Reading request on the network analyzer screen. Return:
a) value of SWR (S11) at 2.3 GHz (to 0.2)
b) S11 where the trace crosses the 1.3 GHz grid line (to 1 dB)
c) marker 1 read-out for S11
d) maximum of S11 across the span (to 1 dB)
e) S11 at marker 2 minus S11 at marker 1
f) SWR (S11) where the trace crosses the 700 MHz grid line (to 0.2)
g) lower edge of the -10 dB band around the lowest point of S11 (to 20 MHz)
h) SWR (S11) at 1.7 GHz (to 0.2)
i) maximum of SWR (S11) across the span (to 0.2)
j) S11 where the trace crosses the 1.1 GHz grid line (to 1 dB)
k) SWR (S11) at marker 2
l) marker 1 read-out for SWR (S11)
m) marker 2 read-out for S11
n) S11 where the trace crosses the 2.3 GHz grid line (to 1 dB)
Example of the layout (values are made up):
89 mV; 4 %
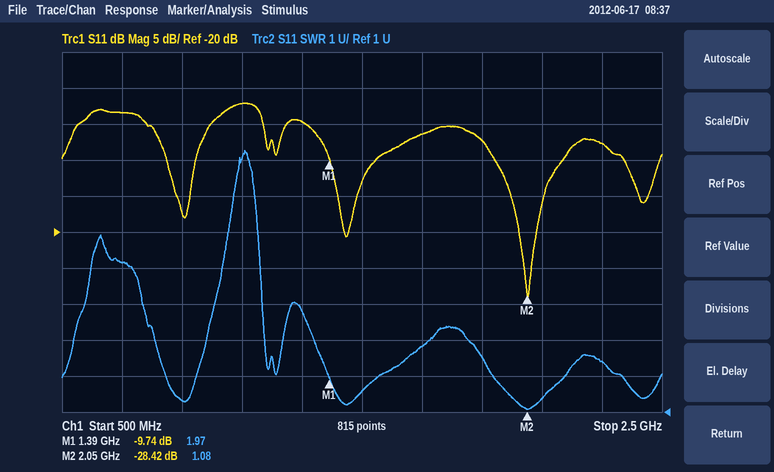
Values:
2.4; -5 dB; -9.74 dB; -2 dB; -18.68 dB; 5.2; 1.94 GHz; 2.8; 8.2; -2 dB; 1.08; 1.97; -28.42 dB; -8 dB
